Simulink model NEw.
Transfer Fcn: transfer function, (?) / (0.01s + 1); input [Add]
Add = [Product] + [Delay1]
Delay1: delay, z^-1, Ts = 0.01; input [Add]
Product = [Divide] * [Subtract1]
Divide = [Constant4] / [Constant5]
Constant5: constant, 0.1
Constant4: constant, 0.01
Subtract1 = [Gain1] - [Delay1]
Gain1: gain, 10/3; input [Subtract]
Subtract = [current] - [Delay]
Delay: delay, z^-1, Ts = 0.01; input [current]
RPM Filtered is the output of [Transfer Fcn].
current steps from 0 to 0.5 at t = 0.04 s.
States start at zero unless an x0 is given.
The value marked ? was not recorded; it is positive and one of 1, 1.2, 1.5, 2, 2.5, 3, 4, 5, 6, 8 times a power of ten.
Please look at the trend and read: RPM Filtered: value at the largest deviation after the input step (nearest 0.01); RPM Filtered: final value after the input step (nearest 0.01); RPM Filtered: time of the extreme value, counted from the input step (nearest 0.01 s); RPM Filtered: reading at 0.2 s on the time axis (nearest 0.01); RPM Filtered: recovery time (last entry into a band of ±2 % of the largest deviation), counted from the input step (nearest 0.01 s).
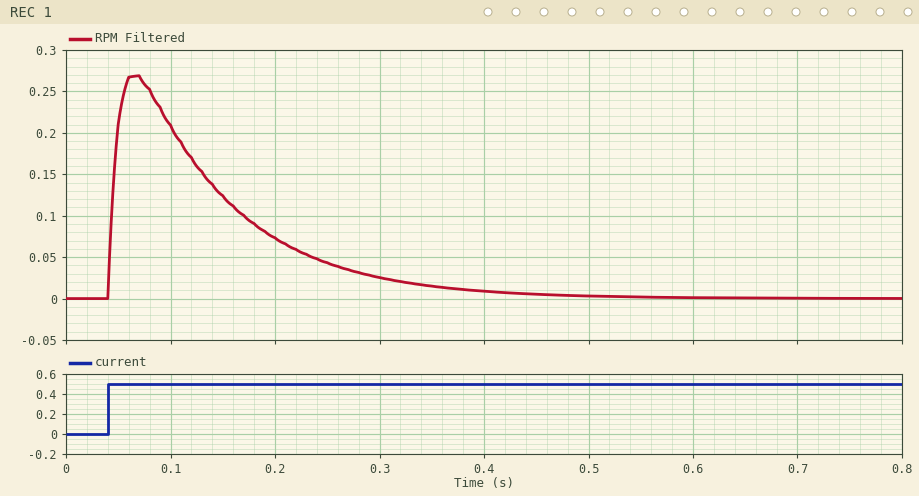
0.27
0.00
0.03 s
0.07
0.41 s
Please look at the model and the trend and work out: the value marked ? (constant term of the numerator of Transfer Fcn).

2
